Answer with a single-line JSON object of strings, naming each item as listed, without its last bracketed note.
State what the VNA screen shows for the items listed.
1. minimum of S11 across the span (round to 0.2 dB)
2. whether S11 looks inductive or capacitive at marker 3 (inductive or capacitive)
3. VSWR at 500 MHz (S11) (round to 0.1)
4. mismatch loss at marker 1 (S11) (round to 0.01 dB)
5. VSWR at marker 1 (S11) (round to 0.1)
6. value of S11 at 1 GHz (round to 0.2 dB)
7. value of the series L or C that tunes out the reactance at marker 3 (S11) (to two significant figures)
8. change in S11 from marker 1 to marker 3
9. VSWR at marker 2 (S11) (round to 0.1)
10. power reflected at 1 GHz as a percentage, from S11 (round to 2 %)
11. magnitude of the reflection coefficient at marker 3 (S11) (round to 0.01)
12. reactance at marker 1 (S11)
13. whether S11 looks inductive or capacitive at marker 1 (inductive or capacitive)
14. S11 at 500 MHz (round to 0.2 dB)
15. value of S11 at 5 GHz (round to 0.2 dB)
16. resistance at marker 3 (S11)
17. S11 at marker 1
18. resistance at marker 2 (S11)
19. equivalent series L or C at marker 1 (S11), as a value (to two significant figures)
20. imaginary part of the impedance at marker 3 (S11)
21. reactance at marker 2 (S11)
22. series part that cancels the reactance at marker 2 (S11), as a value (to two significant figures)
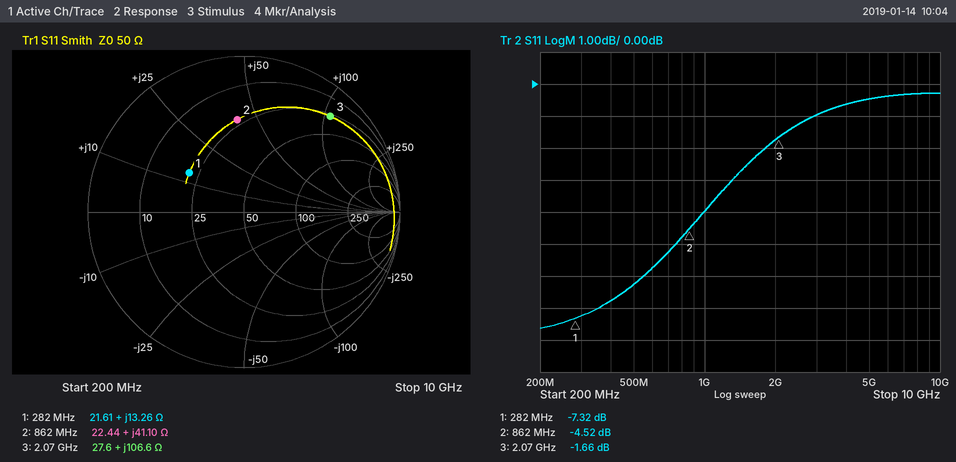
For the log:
{"minimum of S11 across the span": "-7.6 dB", "whether S11 looks inductive or capacitive at marker 3": "inductive", "VSWR at 500 MHz (S11)": "2.9", "mismatch loss at marker 1 (S11)": "0.89 dB", "VSWR at marker 1 (S11)": "2.5", "value of S11 at 1 GHz": "-4.0 dB", "value of the series L or C that tunes out the reactance at marker 3 (S11)": "720 fF", "change in S11 from marker 1 to marker 3": "5.66 dB", "VSWR at marker 2 (S11)": "3.9", "power reflected at 1 GHz as a percentage, from S11": "40 %", "magnitude of the reflection coefficient at marker 3 (S11)": "0.83", "reactance at marker 1": "+13.26 Ω", "whether S11 looks inductive or capacitive at marker 1": "inductive", "S11 at 500 MHz": "-6.2 dB", "value of S11 at 5 GHz": "-0.4 dB", "resistance at marker 3": "27.6 Ω", "S11 at marker 1": "-7.32 dB", "resistance at marker 2": "22.44 Ω", "equivalent series L or C at marker 1 (S11), as a value": "7.5 nH", "imaginary part of the impedance at marker 3": "+106.6 Ω", "reactance at marker 2": "+41.10 Ω", "series part that cancels the reactance at marker 2 (S11), as a value": "4.5 pF"}
